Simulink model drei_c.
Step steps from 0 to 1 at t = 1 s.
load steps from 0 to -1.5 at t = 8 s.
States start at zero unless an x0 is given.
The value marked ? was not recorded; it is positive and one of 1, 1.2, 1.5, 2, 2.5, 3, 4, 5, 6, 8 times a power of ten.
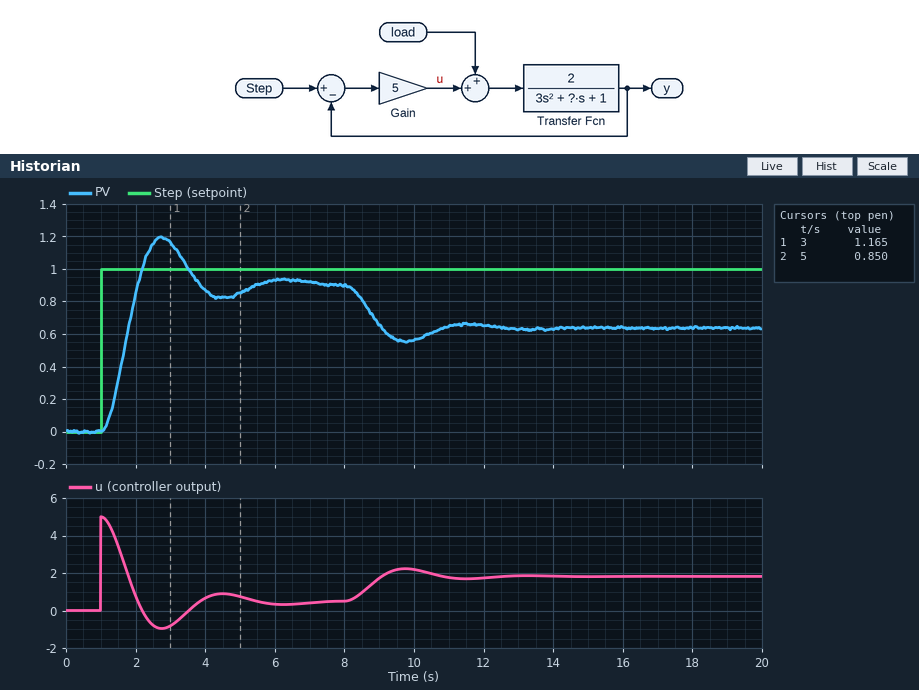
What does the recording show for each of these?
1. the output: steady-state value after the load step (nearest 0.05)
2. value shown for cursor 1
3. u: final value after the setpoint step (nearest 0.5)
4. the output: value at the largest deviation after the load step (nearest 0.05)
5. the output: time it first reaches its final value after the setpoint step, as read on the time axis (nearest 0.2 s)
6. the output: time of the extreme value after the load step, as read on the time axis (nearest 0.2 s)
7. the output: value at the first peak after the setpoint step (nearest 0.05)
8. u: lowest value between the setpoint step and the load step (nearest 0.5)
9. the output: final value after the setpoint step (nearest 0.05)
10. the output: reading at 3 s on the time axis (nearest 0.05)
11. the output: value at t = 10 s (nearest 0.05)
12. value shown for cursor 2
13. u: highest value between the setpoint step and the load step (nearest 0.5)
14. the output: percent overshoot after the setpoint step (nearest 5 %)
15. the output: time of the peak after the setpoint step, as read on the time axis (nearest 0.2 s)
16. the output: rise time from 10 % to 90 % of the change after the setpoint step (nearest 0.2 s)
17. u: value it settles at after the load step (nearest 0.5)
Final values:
0.65
1.165
0.5
0.55
2.0 s
9.8 s
1.20
-1.0
0.90
1.15
0.55
0.850
5.0
30 %
2.8 s
0.8 s
2.0
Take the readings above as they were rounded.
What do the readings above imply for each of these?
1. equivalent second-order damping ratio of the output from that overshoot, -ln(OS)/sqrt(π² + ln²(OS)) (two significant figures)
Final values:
0.36
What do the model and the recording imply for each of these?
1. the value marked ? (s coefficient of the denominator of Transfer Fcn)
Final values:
4
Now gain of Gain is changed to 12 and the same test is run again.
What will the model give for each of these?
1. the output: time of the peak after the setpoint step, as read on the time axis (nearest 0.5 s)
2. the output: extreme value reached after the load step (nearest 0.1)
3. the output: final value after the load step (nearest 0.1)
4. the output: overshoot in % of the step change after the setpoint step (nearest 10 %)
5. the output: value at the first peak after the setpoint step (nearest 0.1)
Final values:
2.0 s
0.8
0.8
50 %
1.4
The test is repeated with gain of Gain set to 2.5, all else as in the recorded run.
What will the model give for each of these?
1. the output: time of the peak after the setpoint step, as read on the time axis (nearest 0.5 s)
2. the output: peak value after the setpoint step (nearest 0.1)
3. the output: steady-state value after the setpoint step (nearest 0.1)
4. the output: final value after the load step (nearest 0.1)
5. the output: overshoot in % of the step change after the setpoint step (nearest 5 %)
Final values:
3.5 s
1.0
0.8
0.3
20 %
